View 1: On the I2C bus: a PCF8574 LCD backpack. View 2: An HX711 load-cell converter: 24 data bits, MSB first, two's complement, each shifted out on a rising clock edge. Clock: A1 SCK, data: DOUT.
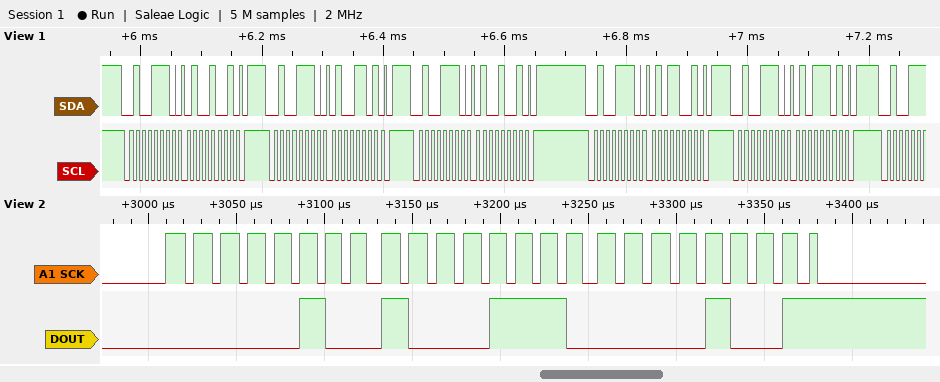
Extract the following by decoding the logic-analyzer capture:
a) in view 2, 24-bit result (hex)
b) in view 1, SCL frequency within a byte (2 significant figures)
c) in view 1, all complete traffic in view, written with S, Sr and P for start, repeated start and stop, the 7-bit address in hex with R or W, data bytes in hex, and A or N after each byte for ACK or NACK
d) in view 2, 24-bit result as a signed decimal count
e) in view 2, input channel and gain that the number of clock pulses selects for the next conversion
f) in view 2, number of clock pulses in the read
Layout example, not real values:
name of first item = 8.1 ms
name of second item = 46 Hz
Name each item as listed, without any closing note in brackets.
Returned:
in view 2, 24-bit result = 0x048E09
in view 1, SCL frequency within a byte = 100 kHz
in view 1, all complete traffic in view, written with S, Sr and P for start, repeated start and stop, the 7-bit address in hex with R or W, data bytes in hex, and A or N after each byte for ACK or NACK = S 27W A 49 A P S 27W A 4D A P S 27W A 49 A P S 27W A 59 A P S 27W A 5D A P
in view 2, 24-bit result as a signed decimal count = 298505
in view 2, input channel and gain that the number of clock pulses selects for the next conversion = channel A, gain 128
in view 2, number of clock pulses in the read = 25
